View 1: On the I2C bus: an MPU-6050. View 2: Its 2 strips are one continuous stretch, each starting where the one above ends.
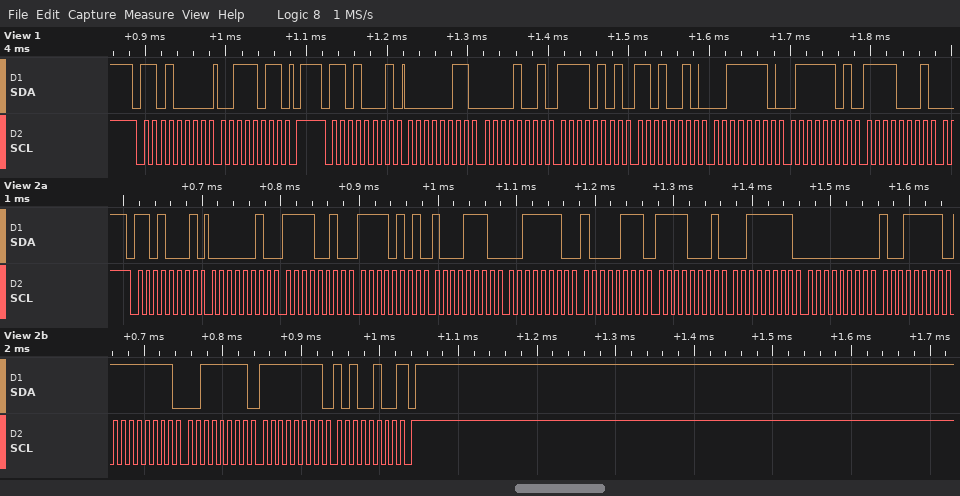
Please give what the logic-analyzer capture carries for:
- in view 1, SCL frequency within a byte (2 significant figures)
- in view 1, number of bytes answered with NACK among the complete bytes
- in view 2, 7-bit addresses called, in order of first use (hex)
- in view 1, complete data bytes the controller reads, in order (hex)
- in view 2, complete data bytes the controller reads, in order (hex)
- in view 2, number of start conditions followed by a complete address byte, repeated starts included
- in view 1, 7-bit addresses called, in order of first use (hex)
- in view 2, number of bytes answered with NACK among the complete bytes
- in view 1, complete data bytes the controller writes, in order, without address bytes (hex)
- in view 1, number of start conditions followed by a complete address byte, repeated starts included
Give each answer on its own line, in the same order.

100 kHz
0
0x68
03 09 F5 D2 3E 7D F1
02 F2 F5 8E 3E 87 F1 3F 00 9F FF 3F FF A4
1
0x68
1
3B
2
